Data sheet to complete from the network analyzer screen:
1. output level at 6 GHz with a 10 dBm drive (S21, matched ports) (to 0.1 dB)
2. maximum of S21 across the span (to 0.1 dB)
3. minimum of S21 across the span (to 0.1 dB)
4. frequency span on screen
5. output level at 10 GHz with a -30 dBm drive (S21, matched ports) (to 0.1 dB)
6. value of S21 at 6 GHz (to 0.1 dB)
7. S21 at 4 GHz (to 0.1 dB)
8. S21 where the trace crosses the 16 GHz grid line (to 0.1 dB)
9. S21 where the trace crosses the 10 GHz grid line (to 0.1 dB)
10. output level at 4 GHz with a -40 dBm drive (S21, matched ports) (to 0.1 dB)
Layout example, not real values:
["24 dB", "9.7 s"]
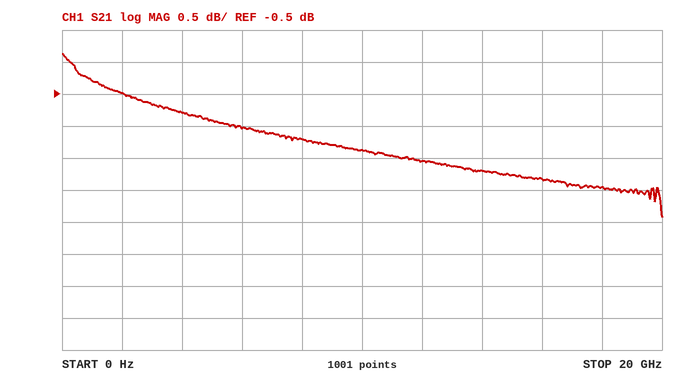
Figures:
["9.0 dBm", "0.1 dB", "-2.4 dB", "20 GHz", "-31.4 dBm", "-1.0 dB", "-0.8 dB", "-1.8 dB", "-1.4 dB", "-40.8 dBm"]
